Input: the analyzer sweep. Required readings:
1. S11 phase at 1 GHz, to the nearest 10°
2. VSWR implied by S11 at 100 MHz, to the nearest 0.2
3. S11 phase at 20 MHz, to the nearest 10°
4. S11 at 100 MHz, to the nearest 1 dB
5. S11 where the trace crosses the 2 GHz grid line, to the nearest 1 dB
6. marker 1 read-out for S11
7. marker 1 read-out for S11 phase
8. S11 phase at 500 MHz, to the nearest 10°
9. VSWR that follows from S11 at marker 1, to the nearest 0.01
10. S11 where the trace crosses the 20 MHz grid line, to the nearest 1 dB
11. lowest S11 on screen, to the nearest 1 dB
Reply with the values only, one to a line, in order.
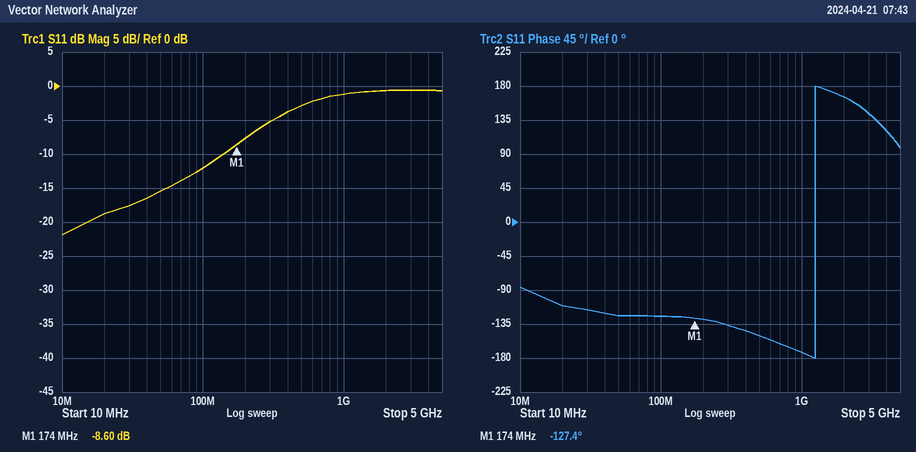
-170°
1.6
-110°
-12 dB
-1 dB
-8.60 dB
-127.4°
-150°
2.18
-19 dB
-22 dB
